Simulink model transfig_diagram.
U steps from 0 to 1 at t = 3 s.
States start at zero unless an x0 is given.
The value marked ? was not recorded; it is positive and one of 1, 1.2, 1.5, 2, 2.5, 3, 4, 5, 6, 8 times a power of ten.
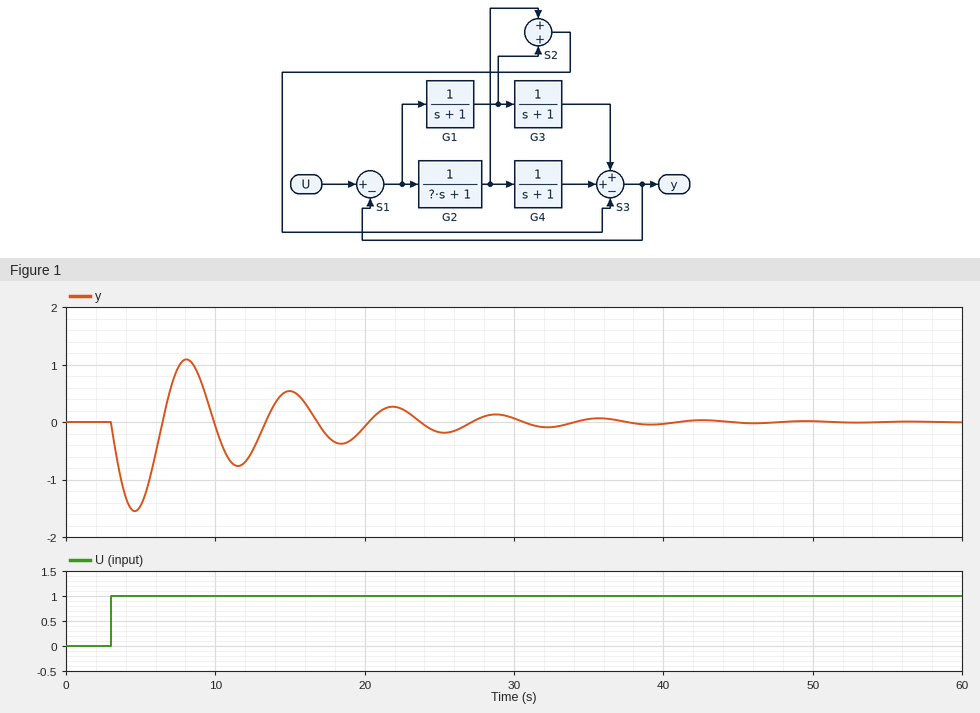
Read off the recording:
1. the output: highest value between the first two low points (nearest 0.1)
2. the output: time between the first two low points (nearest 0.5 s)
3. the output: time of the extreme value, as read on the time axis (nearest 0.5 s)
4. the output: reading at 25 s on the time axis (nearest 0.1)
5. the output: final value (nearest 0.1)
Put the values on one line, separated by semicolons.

1.1; 7.0 s; 4.5 s; -0.2; 0.0
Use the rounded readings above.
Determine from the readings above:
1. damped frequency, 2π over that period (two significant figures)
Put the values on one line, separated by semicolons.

0.90 rad/s
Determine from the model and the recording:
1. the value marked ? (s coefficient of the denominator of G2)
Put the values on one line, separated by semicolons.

1.5
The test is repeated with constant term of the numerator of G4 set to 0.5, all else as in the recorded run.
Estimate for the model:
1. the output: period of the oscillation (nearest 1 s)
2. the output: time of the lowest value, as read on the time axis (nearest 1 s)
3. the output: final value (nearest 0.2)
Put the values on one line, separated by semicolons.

9 s; 6 s; -1.0
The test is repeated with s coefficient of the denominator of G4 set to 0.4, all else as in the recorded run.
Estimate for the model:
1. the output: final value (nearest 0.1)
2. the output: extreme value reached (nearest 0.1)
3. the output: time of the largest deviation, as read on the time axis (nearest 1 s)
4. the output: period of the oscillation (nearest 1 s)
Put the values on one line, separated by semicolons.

0.0; -1.0; 4 s; 6 s
